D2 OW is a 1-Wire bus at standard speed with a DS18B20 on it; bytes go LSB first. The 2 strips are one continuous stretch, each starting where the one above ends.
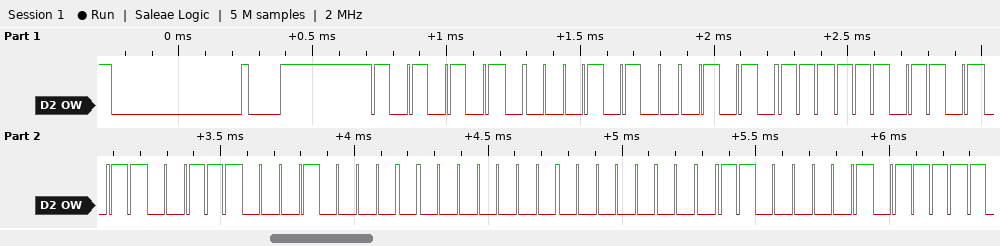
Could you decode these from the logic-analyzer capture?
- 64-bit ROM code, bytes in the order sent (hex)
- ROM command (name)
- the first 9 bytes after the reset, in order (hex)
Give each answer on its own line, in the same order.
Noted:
28 EA B7 E6 08 00 00 83
Match ROM
55 28 EA B7 E6 08 00 00 83
